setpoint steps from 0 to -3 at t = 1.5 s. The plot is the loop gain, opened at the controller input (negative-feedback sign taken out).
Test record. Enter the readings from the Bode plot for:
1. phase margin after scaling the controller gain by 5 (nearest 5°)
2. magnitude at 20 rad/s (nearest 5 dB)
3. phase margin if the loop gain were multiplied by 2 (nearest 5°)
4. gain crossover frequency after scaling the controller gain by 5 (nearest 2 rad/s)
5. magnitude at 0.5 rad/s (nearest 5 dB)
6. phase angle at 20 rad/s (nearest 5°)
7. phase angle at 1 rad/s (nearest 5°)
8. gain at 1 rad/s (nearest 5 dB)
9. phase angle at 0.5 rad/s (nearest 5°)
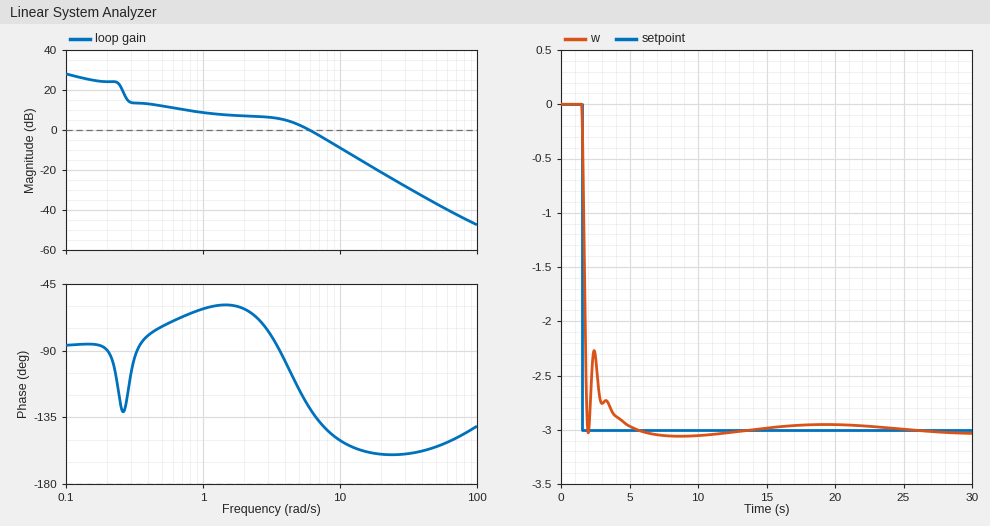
25°
-20 dB
35°
14 rad/s
10 dB
-160°
-60°
10 dB
-75°
